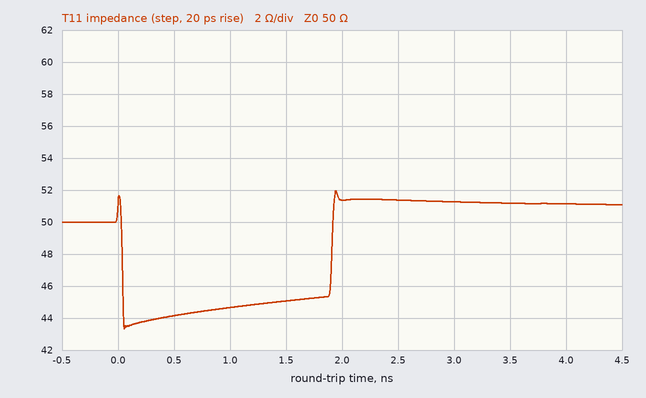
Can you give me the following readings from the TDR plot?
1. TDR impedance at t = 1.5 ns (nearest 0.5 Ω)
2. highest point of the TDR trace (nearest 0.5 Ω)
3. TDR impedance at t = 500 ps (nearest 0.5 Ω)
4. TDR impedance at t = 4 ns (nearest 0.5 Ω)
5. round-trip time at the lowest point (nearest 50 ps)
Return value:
45.0 Ω
52.0 Ω
44.0 Ω
51.0 Ω
50 ps
